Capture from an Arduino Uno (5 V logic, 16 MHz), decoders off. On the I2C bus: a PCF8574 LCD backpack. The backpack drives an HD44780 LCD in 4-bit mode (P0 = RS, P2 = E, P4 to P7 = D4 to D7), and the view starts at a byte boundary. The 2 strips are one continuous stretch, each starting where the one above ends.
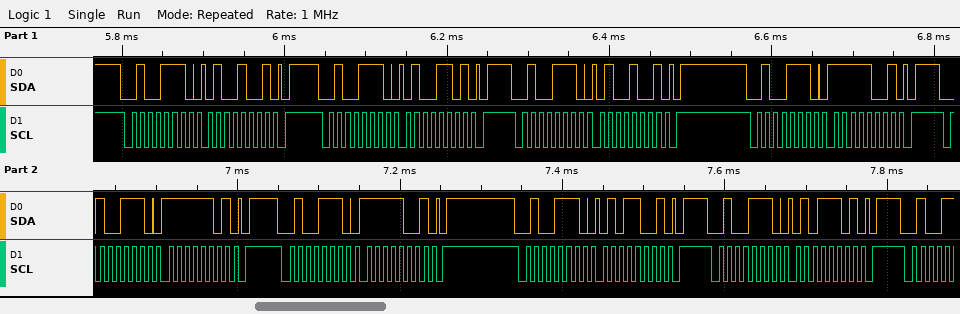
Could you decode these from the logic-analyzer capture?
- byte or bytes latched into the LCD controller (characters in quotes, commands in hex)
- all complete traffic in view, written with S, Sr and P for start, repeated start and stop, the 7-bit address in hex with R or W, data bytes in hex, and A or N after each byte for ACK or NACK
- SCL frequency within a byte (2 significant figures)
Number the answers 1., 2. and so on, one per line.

1. 'O'
2. S 27W A 49 A P S 27W A 4D A P S 27W A 49 A P S 27W A F9 A P S 27W A FD A P S 27W A F9 A P S 27W A 59 A P S 27W A 5D A P
3. 100 kHz
